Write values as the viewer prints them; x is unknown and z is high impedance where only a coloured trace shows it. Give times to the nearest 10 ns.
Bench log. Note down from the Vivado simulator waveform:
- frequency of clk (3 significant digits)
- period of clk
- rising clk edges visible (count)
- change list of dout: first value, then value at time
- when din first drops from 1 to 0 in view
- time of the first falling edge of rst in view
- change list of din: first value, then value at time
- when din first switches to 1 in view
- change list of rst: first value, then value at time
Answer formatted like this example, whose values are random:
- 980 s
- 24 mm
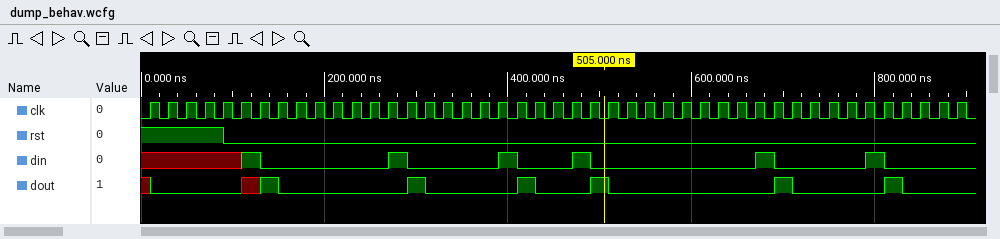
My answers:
- 50.0 MHz
- 20 ns
- 45
- x, 0 at 10 ns, x at 110 ns, 1 at 130 ns, 0 at 150 ns, 1 at 290 ns, 0 at 310 ns, 1 at 410 ns, 0 at 430 ns, 1 at 490 ns, 0 at 510 ns, 1 at 690 ns, 0 at 710 ns, 1 at 810 ns, 0 at 830 ns
- 130 ns
- 90 ns
- x, 1 at 110 ns, 0 at 130 ns, 1 at 270 ns, 0 at 290 ns, 1 at 390 ns, 0 at 410 ns, 1 at 470 ns, 0 at 490 ns, 1 at 670 ns, 0 at 690 ns, 1 at 790 ns, 0 at 810 ns
- 110 ns
- 1, 0 at 90 ns
